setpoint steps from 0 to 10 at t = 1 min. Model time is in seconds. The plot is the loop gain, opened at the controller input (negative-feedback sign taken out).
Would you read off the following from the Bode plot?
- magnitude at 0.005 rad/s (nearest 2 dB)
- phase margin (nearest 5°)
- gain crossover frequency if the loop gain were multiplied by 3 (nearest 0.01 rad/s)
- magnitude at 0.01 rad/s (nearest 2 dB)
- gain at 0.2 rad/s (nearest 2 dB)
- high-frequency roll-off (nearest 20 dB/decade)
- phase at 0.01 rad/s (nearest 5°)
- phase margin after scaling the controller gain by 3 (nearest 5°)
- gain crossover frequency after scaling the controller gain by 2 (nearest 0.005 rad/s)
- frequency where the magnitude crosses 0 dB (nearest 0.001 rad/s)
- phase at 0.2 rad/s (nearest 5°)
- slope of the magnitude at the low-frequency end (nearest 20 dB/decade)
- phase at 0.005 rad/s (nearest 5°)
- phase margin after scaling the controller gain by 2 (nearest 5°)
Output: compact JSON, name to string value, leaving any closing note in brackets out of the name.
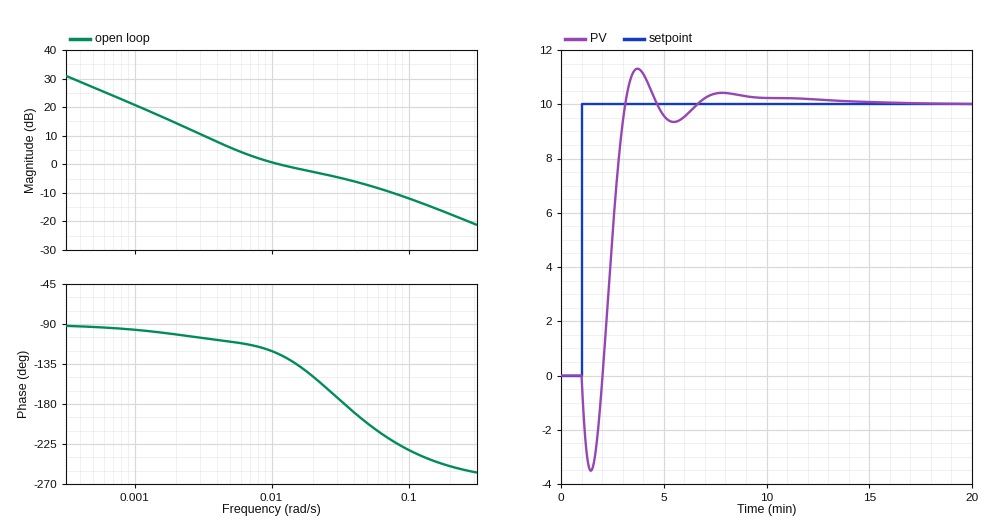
{"magnitude at 0.005 rad/s": "6 dB", "phase margin": "55°", "gain crossover frequency if the loop gain were multiplied by 3": "0.07 rad/s", "magnitude at 0.01 rad/s": "0 dB", "gain at 0.2 rad/s": "-18 dB", "high-frequency roll-off": "-20 dB/decade", "phase at 0.01 rad/s": "-120°", "phase margin after scaling the controller gain by 3": "-40°", "gain crossover frequency after scaling the controller gain by 2": "0.040 rad/s", "frequency where the magnitude crosses 0 dB": "0.011 rad/s", "phase at 0.2 rad/s": "-250°", "slope of the magnitude at the low-frequency end": "-20 dB/decade", "phase at 0.005 rad/s": "-110°", "phase margin after scaling the controller gain by 2": "-10°"}
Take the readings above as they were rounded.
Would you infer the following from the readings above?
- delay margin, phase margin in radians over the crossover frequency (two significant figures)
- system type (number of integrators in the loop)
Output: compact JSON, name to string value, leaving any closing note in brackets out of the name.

{"delay margin, phase margin in radians over the crossover frequency": "87 s", "system type": "1"}
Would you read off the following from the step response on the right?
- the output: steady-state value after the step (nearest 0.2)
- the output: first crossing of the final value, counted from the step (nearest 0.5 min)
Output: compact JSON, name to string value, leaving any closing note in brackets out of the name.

{"the output: steady-state value after the step": "10.0", "the output: first crossing of the final value, counted from the step": "2.0 min"}
